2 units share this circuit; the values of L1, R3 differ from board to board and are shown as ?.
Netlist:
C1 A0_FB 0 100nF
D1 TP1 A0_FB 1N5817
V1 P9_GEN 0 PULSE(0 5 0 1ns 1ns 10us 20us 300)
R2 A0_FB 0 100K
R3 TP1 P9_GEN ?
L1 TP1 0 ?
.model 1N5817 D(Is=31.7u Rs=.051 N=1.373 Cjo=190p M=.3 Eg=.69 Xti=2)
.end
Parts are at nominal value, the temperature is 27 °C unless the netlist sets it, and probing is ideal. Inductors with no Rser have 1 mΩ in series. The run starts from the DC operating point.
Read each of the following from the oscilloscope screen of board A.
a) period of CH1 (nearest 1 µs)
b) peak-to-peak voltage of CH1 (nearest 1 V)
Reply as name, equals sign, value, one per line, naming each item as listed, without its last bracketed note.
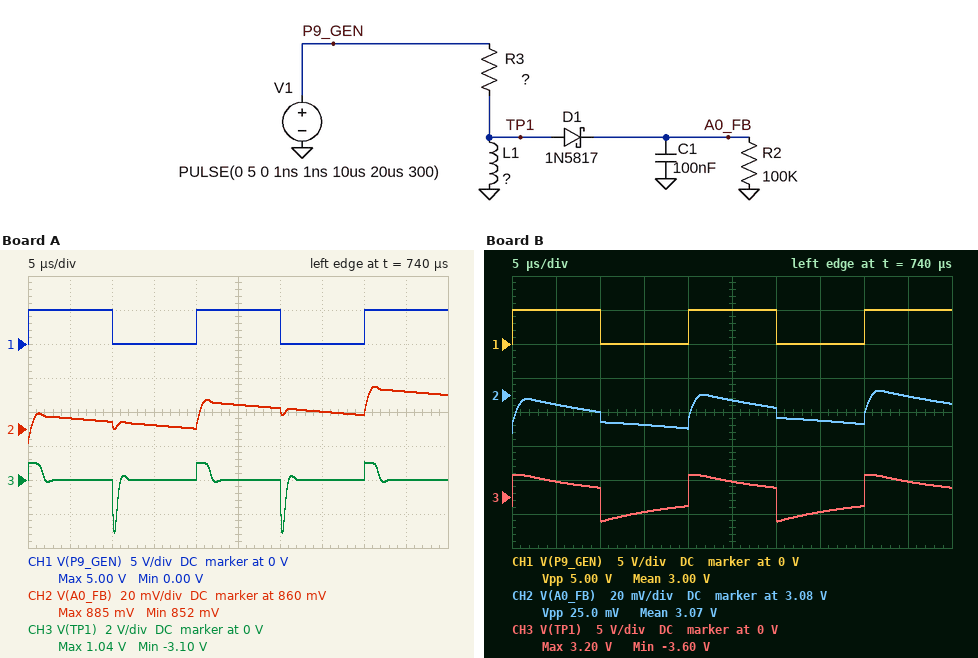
period of CH1 = 20 µs
peak-to-peak voltage of CH1 = 5 V
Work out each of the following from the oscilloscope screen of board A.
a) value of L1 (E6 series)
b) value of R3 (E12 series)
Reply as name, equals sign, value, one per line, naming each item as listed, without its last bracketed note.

value of L1 = 470 µH
value of R3 = 1.5 kΩ
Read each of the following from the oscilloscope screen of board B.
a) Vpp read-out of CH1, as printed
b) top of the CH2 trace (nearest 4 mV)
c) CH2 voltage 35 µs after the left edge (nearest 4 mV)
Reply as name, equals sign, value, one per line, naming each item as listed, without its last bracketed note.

Vpp read-out of CH1, as printed = 5.00 V
top of the CH2 trace = 3.084 V
CH2 voltage 35 µs after the left edge = 3.064 V
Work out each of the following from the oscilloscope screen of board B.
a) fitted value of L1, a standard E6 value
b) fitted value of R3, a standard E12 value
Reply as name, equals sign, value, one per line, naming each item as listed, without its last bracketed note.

fitted value of L1, a standard E6 value = 2.2 mH
fitted value of R3, a standard E12 value = 220 Ω
